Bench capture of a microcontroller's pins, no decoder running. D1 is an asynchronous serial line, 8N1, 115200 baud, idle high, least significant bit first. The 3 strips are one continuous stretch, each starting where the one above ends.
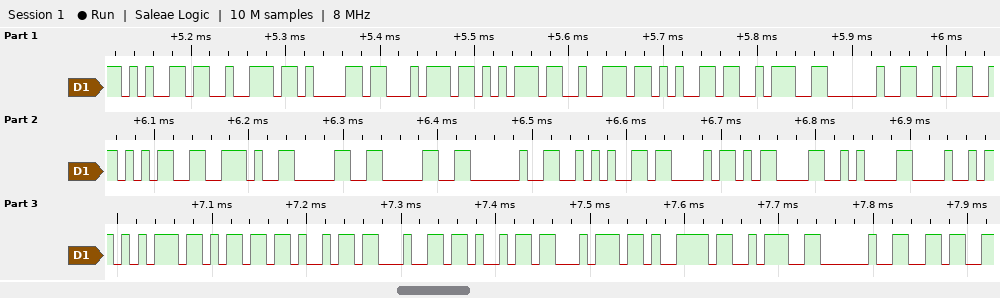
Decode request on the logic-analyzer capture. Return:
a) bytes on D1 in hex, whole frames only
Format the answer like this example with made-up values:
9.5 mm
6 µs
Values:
65 72 61 74 75 72 65 3A 20 32 35 2E 30 30 20 2A 43 0D 0A 48 75 6D 69 64 69 74 79 3A 20 36
